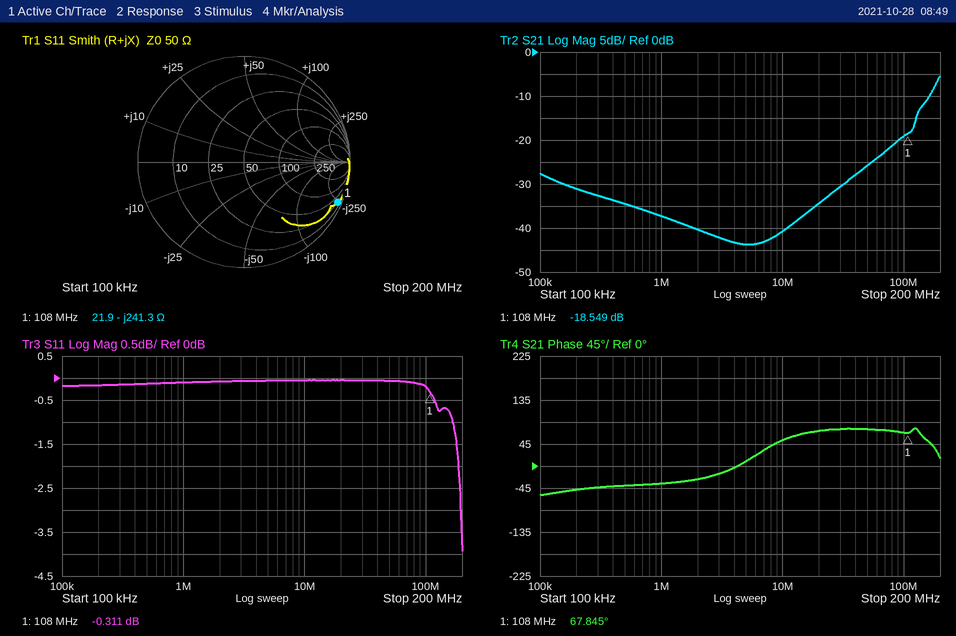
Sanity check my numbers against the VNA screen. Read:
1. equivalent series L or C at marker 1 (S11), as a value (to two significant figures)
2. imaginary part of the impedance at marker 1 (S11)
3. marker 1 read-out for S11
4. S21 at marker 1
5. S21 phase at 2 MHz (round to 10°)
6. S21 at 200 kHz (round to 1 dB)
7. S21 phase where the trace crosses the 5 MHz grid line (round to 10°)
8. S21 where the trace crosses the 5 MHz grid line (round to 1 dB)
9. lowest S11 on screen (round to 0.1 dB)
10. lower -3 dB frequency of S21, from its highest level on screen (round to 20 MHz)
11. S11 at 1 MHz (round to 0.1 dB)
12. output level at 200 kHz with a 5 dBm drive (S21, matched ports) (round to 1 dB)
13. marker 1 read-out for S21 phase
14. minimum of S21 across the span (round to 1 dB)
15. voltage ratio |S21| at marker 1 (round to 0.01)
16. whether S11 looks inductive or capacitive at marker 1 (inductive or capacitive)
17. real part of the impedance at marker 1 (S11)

6.1 pF
-241.3 Ω
-0.311 dB
-18.549 dB
-30°
-31 dB
10°
-44 dB
-3.9 dB
180 MHz
-0.1 dB
-26 dBm
67.845°
-44 dB
0.12
capacitive
21.9 Ω
